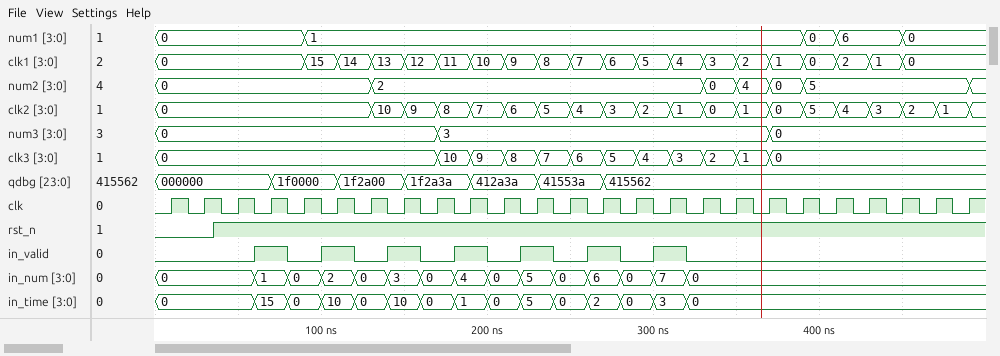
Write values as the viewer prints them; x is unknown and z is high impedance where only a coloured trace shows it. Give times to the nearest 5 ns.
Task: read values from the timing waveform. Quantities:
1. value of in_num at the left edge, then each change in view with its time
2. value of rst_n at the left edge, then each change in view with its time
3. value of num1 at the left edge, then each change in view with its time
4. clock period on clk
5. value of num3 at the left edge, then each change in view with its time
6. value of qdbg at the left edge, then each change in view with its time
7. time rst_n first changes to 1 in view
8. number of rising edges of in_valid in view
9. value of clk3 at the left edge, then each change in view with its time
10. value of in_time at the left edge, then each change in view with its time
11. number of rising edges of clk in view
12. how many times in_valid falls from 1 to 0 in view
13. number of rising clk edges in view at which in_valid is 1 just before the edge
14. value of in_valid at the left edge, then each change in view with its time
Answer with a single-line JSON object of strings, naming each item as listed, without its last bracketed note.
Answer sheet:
{"value of in_num at the left edge, then each change in view with its time": "0, 1 at 60 ns, 0 at 80 ns, 2 at 100 ns, 0 at 120 ns, 3 at 140 ns, 0 at 160 ns, 4 at 180 ns, 0 at 200 ns, 5 at 220 ns, 0 at 240 ns, 6 at 260 ns, 0 at 280 ns, 7 at 300 ns, 0 at 320 ns", "value of rst_n at the left edge, then each change in view with its time": "0, 1 at 35 ns", "value of num1 at the left edge, then each change in view with its time": "0, 1 at 90 ns, 0 at 390 ns, 6 at 410 ns, 0 at 450 ns", "clock period on clk": "20 ns", "value of num3 at the left edge, then each change in view with its time": "0, 3 at 170 ns, 0 at 370 ns", "value of qdbg at the left edge, then each change in view with its time": "000000, 1f0000 at 70 ns, 1f2a00 at 110 ns, 1f2a3a at 150 ns, 412a3a at 190 ns, 41553a at 230 ns, 415562 at 270 ns", "time rst_n first changes to 1 in view": "35 ns", "number of rising edges of in_valid in view": "7", "value of clk3 at the left edge, then each change in view with its time": "0, 10 at 170 ns, 9 at 190 ns, 8 at 210 ns, 7 at 230 ns, 6 at 250 ns, 5 at 270 ns, 4 at 290 ns, 3 at 310 ns, 2 at 330 ns, 1 at 350 ns, 0 at 370 ns", "value of in_time at the left edge, then each change in view with its time": "0, 15 at 60 ns, 0 at 80 ns, 10 at 100 ns, 0 at 120 ns, 10 at 140 ns, 0 at 160 ns, 1 at 180 ns, 0 at 200 ns, 5 at 220 ns, 0 at 240 ns, 2 at 260 ns, 0 at 280 ns, 3 at 300 ns, 0 at 320 ns", "number of rising edges of clk in view": "25", "how many times in_valid falls from 1 to 0 in view": "7", "number of rising clk edges in view at which in_valid is 1 just before the edge": "7", "value of in_valid at the left edge, then each change in view with its time": "0, 1 at 60 ns, 0 at 80 ns, 1 at 100 ns, 0 at 120 ns, 1 at 140 ns, 0 at 160 ns, 1 at 180 ns, 0 at 200 ns, 1 at 220 ns, 0 at 240 ns, 1 at 260 ns, 0 at 280 ns, 1 at 300 ns, 0 at 320 ns"}
